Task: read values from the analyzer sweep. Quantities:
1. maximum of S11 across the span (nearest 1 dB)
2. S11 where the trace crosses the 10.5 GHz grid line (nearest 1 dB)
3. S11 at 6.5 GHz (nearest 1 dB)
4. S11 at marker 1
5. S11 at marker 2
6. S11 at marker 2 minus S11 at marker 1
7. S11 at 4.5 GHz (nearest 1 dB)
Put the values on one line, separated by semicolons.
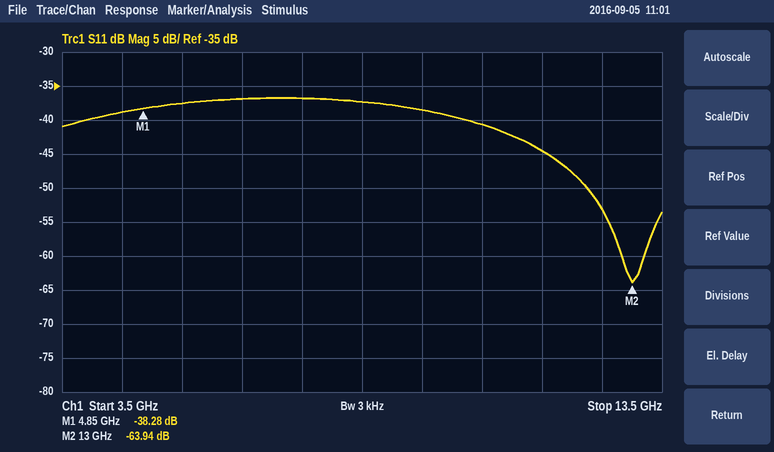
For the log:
-37 dB; -41 dB; -37 dB; -38.28 dB; -63.94 dB; -25.66 dB; -39 dB
